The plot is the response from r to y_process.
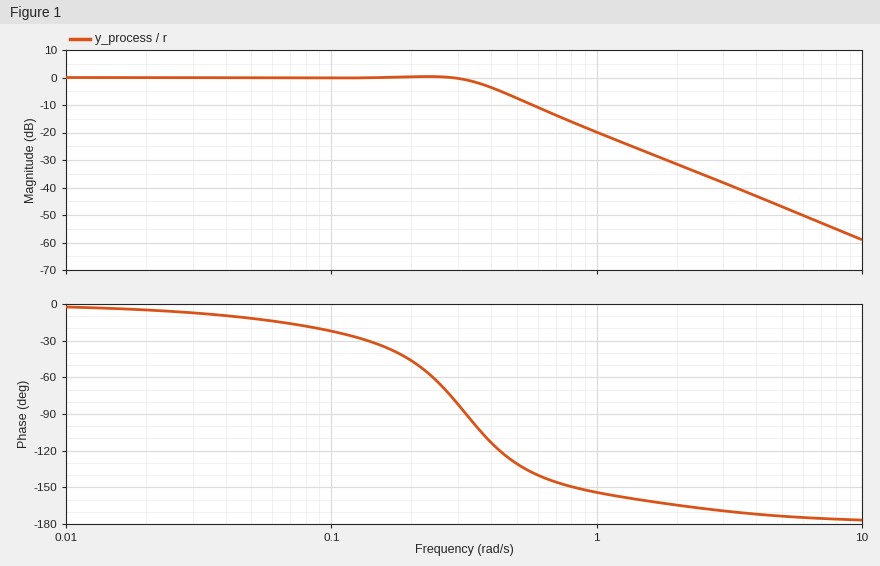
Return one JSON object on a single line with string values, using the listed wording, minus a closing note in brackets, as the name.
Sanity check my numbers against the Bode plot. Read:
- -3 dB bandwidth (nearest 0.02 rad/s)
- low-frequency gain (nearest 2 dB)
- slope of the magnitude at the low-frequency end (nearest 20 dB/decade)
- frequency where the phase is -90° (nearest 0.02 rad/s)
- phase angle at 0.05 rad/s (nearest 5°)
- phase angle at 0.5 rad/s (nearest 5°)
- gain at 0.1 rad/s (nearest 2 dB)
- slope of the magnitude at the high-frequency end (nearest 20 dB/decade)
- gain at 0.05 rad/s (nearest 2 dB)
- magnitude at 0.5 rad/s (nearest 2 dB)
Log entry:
{"-3 dB bandwidth": "0.38 rad/s", "low-frequency gain": "0 dB", "slope of the magnitude at the low-frequency end": "0 dB/decade", "frequency where the phase is -90°": "0.32 rad/s", "phase angle at 0.05 rad/s": "-10°", "phase angle at 0.5 rad/s": "-130°", "gain at 0.1 rad/s": "0 dB", "slope of the magnitude at the high-frequency end": "-40 dB/decade", "gain at 0.05 rad/s": "0 dB", "magnitude at 0.5 rad/s": "-8 dB"}
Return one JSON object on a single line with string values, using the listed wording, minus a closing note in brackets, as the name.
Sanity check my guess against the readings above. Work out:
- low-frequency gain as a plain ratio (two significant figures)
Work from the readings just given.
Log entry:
{"low-frequency gain as a plain ratio": "1.0"}
